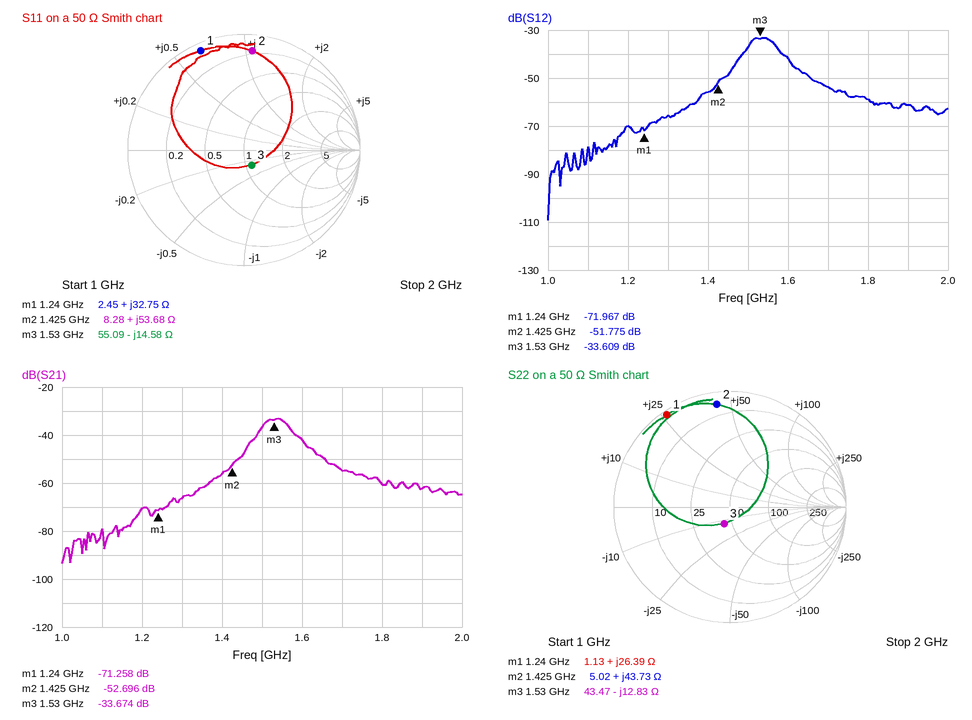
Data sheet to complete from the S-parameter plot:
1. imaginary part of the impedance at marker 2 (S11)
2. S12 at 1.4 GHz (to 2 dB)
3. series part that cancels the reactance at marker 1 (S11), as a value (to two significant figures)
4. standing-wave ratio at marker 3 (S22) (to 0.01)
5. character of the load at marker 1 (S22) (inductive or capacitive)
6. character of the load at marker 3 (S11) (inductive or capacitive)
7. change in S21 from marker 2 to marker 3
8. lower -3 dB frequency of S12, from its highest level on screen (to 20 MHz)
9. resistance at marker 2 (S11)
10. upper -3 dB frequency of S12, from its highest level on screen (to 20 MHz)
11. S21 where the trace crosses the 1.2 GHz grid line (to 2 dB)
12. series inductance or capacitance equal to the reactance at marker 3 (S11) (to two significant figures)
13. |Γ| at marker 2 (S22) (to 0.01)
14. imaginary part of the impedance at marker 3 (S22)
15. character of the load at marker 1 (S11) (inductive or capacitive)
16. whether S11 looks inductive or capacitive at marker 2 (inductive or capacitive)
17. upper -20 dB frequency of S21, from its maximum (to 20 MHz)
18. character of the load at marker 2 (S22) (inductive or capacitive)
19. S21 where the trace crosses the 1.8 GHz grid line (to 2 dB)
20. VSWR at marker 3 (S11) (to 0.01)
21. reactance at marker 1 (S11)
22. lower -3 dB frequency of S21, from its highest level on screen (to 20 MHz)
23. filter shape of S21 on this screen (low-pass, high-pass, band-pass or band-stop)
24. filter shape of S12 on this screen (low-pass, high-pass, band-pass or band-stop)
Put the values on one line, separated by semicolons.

+53.68 Ω; -56 dB; 3.9 pF; 1.36; inductive; capacitive; 19.022 dB; 1.50 GHz; 8.28 Ω; 1.56 GHz; -70 dB; 7.1 pF; 0.89; -12.83 Ω; inductive; inductive; 1.68 GHz; inductive; -60 dB; 1.34; +32.75 Ω; 1.50 GHz; band-pass; band-pass
